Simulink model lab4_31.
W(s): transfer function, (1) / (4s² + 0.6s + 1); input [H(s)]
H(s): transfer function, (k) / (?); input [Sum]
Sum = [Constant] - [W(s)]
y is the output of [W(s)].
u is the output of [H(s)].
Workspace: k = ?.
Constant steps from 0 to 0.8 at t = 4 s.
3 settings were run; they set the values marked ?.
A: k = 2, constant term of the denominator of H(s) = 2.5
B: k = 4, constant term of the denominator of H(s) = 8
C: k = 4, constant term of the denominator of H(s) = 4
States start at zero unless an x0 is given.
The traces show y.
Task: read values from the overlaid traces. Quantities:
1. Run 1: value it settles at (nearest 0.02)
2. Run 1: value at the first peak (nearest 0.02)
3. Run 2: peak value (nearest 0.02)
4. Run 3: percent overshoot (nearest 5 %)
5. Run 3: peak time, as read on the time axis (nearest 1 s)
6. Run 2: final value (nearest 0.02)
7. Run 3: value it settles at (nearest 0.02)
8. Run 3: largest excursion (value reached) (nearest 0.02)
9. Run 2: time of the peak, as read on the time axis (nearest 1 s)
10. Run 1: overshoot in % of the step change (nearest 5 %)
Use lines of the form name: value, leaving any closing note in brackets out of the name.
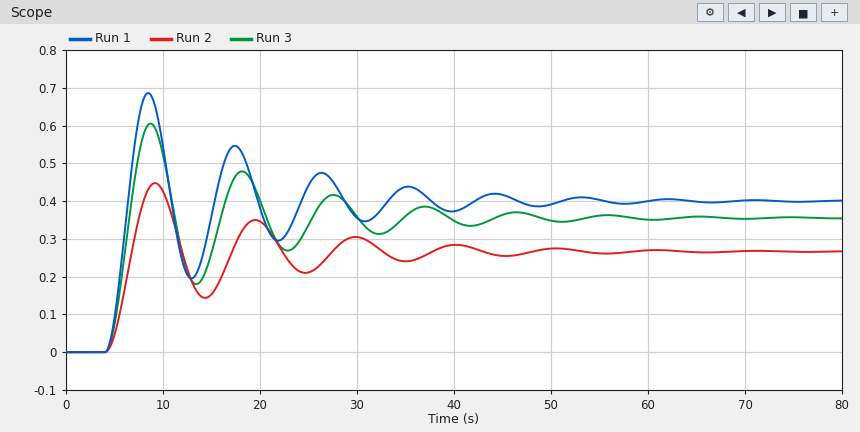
Run 1: value it settles at: 0.40
Run 1: value at the first peak: 0.68
Run 2: peak value: 0.44
Run 3: percent overshoot: 70 %
Run 3: peak time, as read on the time axis: 9 s
Run 2: final value: 0.26
Run 3: value it settles at: 0.36
Run 3: largest excursion (value reached): 0.60
Run 2: time of the peak, as read on the time axis: 9 s
Run 1: overshoot in % of the step change: 70 %
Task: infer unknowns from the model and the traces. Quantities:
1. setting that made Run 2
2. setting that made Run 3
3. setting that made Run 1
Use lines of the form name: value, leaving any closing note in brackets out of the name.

setting that made Run 2: B
setting that made Run 3: A
setting that made Run 1: C
